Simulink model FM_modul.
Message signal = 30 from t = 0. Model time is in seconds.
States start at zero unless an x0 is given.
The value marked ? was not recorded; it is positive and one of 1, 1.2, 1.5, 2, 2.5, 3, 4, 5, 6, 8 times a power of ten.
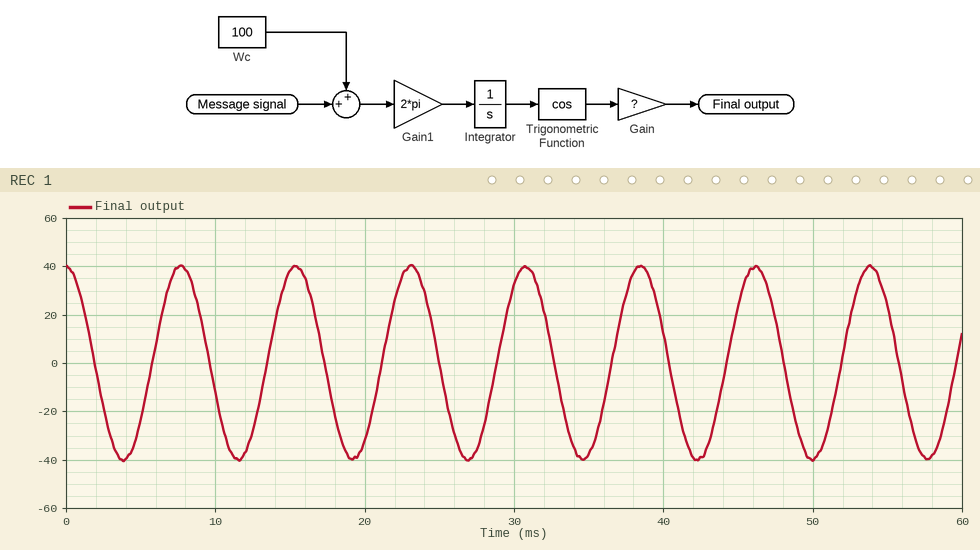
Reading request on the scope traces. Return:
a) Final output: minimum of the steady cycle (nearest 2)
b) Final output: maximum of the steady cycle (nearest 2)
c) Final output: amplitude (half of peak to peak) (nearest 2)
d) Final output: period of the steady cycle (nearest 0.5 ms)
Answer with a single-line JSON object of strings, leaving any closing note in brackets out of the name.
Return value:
{"Final output: minimum of the steady cycle": "-40", "Final output: maximum of the steady cycle": "40", "Final output: amplitude (half of peak to peak)": "40", "Final output: period of the steady cycle": "7.5 ms"}
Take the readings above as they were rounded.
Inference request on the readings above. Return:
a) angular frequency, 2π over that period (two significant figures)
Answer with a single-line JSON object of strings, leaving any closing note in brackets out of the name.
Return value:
{"angular frequency, 2π over that period": "0.84 rad/ms"}
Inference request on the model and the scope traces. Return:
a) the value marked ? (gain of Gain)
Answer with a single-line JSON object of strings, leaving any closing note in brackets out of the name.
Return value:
{"the value marked ?": "40"}
